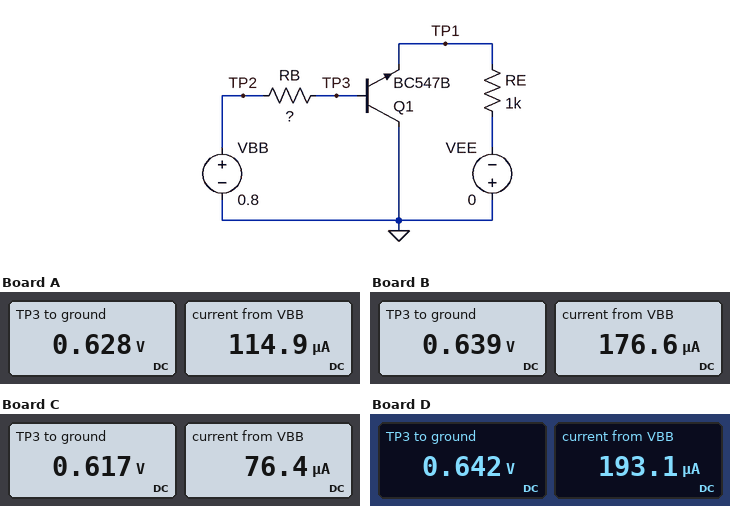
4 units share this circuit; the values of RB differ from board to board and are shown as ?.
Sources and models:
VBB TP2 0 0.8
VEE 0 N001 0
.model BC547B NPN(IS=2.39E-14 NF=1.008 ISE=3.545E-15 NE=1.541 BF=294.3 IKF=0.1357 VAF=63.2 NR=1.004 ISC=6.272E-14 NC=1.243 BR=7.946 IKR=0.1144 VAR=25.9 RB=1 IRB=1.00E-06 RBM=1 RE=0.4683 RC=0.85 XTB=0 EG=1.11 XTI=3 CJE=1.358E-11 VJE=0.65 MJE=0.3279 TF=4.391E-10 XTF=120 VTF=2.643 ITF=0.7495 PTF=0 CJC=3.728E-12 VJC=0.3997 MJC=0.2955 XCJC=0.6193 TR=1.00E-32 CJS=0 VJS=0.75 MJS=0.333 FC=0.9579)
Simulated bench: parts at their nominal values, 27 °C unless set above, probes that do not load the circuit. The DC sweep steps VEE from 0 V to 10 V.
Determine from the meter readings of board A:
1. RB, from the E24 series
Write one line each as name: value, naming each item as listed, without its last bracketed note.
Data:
RB, from the E24 series: 1.5 kΩ
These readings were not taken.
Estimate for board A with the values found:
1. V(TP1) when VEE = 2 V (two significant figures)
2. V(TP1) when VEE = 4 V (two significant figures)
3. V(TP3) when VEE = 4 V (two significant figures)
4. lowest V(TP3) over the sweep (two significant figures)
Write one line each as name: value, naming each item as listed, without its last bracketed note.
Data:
V(TP1) when VEE = 2 V: -41 mV
V(TP1) when VEE = 4 V: -59 mV
V(TP3) when VEE = 4 V: 620 mV
lowest V(TP3) over the sweep: 610 mV
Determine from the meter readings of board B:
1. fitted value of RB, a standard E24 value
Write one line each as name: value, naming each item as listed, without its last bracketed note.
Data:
fitted value of RB, a standard E24 value: 910 Ω
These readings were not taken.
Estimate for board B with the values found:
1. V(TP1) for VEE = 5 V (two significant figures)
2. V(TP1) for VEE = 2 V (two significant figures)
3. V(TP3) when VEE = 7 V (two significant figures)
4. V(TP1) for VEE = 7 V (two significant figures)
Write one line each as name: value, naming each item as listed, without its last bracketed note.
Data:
V(TP1) for VEE = 5 V: -56 mV
V(TP1) for VEE = 2 V: -32 mV
V(TP3) when VEE = 7 V: 630 mV
V(TP1) for VEE = 7 V: -67 mV
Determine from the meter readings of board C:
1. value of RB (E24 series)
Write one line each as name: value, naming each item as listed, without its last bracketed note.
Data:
value of RB: 2.4 kΩ
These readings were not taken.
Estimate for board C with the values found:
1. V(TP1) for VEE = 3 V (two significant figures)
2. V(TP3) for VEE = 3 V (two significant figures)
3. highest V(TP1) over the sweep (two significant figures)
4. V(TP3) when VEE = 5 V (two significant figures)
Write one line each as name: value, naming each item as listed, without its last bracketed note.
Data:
V(TP1) for VEE = 3 V: -61 mV
V(TP3) for VEE = 3 V: 610 mV
highest V(TP1) over the sweep: -2.2 mV
V(TP3) when VEE = 5 V: 610 mV
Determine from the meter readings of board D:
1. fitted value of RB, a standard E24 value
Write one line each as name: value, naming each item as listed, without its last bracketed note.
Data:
fitted value of RB, a standard E24 value: 820 Ω
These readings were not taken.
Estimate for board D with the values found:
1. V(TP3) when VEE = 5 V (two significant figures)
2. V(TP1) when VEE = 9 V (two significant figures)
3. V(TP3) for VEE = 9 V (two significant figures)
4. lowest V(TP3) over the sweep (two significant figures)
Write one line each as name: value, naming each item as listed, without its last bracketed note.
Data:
V(TP3) when VEE = 5 V: 640 mV
V(TP1) when VEE = 9 V: -74 mV
V(TP3) for VEE = 9 V: 630 mV
lowest V(TP3) over the sweep: 630 mV
